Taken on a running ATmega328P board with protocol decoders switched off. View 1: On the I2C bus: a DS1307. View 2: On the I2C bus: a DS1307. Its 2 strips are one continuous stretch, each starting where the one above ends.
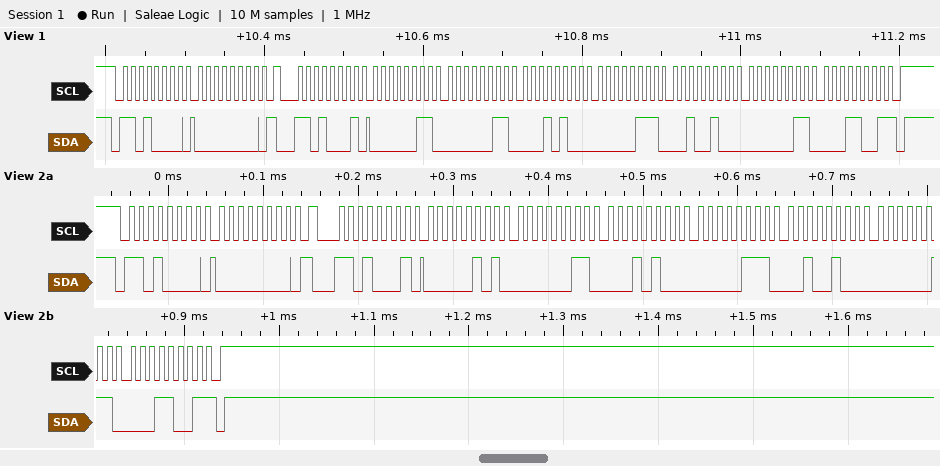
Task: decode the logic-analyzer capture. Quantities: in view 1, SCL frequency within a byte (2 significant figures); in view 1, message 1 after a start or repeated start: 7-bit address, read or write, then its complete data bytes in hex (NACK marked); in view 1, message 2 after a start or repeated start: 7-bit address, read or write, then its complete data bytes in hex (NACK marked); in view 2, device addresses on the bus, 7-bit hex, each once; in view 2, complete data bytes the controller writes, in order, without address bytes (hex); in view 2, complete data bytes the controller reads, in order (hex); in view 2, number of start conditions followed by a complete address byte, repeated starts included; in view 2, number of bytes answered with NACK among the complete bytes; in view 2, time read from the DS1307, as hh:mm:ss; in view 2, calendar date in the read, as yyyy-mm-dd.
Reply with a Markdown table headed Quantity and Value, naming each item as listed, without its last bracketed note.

| Quantity | Value |
|---|---|
| in view 1, SCL frequency within a byte | 100 kHz |
| in view 1, message 1 after a start or repeated start: 7-bit address, read or write, then its complete data bytes in hex | 0x68 write: 00 |
| in view 1, message 2 after a start or repeated start: 7-bit address, read or write, then its complete data bytes in hex | 0x68 read: 03 03 14 07 24 03 19 NACK |
| in view 2, device addresses on the bus, 7-bit hex, each once | 0x68 |
| in view 2, complete data bytes the controller writes, in order, without address bytes | 00 |
| in view 2, complete data bytes the controller reads, in order | 05 03 14 07 24 03 19 |
| in view 2, number of start conditions followed by a complete address byte, repeated starts included | 2 |
| in view 2, number of bytes answered with NACK among the complete bytes | 1 |
| in view 2, time read from the DS1307, as hh:mm:ss | 14:03:05 |
| in view 2, calendar date in the read, as yyyy-mm-dd | 2019-03-24 |
